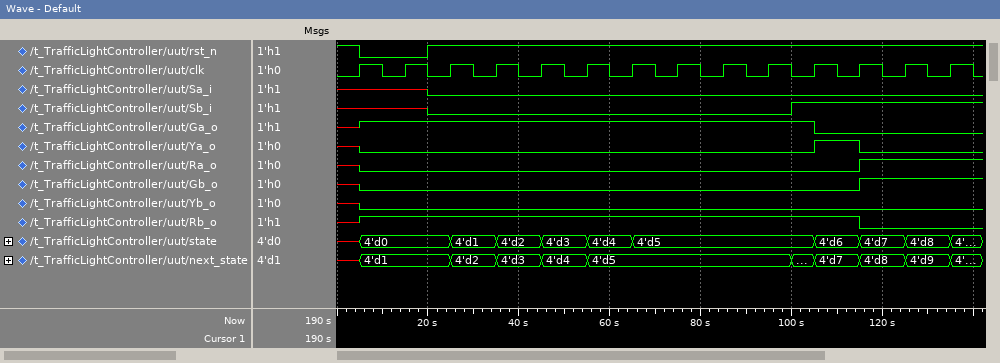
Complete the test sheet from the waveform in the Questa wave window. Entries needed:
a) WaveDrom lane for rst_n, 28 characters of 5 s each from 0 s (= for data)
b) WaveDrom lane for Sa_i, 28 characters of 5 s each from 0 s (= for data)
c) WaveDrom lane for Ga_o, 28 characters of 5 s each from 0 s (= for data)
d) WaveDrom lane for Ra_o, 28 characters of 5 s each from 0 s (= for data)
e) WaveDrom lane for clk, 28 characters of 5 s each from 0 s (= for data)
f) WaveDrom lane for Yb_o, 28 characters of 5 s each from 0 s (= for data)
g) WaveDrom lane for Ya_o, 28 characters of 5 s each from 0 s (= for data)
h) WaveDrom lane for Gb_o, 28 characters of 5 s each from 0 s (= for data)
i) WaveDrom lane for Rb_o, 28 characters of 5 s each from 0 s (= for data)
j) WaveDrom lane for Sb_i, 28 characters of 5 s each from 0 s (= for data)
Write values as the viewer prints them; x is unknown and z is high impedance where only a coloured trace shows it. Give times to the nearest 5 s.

{name: 'rst_n', wave: '10..1.......................'}
{name: 'Sa_i', wave: 'x...0.......................'}
{name: 'Ga_o', wave: 'x1...................0......'}
{name: 'Ra_o', wave: 'x0.....................1....'}
{name: 'clk', wave: '0101010101010101010101010101'}
{name: 'Yb_o', wave: 'x0..........................'}
{name: 'Ya_o', wave: 'x0...................1.0....'}
{name: 'Gb_o', wave: 'x0.....................1....'}
{name: 'Rb_o', wave: 'x1.....................0....'}
{name: 'Sb_i', wave: 'x...0...............1.......'}
